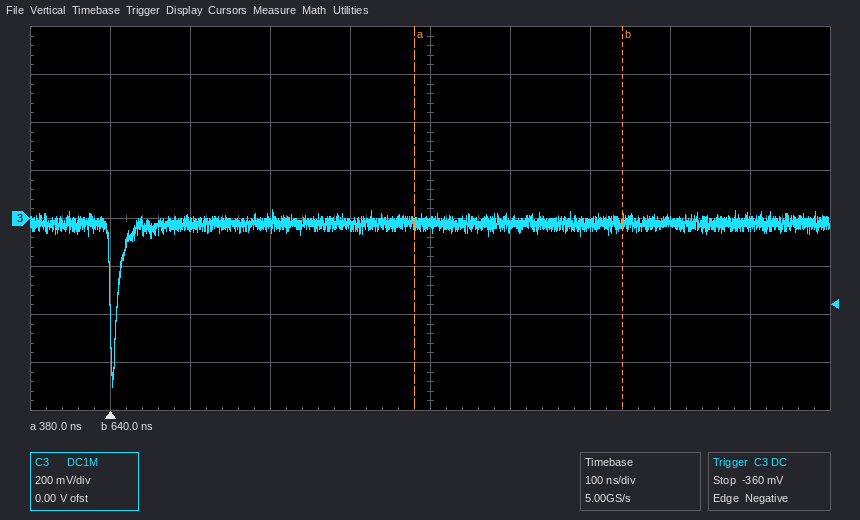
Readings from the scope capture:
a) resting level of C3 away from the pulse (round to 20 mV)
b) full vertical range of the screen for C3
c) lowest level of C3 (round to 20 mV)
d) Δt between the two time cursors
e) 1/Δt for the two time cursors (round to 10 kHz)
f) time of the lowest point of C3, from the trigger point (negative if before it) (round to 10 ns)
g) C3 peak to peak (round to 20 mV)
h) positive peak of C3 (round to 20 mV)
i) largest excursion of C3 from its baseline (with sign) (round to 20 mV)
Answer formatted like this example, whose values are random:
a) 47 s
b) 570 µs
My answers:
a) -20 mV
b) 1.6 V
c) -700 mV
d) 260 ns
e) 3.85 MHz
f) 0 ns
g) 740 mV
h) 40 mV
i) -680 mV
